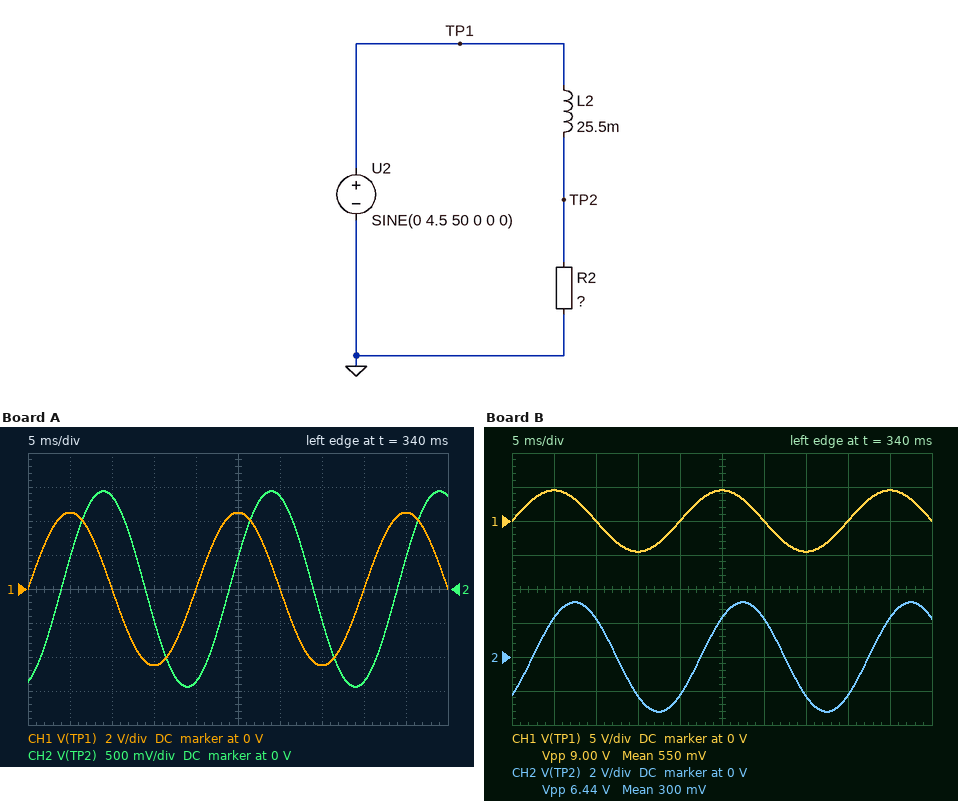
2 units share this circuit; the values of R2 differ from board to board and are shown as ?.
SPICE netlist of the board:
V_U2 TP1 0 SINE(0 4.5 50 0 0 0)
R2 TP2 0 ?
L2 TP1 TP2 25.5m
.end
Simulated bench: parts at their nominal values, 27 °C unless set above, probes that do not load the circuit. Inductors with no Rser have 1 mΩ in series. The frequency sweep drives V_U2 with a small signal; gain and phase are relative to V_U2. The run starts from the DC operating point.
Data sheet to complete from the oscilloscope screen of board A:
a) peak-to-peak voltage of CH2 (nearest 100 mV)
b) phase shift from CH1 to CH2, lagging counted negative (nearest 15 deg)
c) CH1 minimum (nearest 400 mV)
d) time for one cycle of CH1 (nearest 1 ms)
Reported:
2.9 V
-75 deg
-4.4 V
20 ms
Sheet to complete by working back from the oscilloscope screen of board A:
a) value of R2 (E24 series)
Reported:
2.7 Ω
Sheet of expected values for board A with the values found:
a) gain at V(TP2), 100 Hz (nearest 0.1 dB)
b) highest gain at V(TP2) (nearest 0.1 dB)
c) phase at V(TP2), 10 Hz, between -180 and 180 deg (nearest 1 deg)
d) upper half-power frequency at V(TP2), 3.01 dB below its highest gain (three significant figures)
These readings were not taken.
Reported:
-15.6 dB
0 dB
-31 deg
16.9 Hz
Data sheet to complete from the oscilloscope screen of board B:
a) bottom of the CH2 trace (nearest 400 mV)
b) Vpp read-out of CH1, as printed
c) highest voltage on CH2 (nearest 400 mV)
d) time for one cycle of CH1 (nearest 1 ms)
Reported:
-3.2 V
9.00 V
3.2 V
20 ms
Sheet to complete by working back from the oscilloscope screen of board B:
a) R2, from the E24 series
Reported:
8.2 Ω
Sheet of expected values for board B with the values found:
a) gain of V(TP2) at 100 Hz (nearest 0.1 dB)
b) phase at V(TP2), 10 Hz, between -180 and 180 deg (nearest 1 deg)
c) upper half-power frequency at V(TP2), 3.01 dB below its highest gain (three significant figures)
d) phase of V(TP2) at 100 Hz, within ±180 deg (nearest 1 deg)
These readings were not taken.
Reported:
-6.8 dB
-11 deg
51.2 Hz
-63 deg
